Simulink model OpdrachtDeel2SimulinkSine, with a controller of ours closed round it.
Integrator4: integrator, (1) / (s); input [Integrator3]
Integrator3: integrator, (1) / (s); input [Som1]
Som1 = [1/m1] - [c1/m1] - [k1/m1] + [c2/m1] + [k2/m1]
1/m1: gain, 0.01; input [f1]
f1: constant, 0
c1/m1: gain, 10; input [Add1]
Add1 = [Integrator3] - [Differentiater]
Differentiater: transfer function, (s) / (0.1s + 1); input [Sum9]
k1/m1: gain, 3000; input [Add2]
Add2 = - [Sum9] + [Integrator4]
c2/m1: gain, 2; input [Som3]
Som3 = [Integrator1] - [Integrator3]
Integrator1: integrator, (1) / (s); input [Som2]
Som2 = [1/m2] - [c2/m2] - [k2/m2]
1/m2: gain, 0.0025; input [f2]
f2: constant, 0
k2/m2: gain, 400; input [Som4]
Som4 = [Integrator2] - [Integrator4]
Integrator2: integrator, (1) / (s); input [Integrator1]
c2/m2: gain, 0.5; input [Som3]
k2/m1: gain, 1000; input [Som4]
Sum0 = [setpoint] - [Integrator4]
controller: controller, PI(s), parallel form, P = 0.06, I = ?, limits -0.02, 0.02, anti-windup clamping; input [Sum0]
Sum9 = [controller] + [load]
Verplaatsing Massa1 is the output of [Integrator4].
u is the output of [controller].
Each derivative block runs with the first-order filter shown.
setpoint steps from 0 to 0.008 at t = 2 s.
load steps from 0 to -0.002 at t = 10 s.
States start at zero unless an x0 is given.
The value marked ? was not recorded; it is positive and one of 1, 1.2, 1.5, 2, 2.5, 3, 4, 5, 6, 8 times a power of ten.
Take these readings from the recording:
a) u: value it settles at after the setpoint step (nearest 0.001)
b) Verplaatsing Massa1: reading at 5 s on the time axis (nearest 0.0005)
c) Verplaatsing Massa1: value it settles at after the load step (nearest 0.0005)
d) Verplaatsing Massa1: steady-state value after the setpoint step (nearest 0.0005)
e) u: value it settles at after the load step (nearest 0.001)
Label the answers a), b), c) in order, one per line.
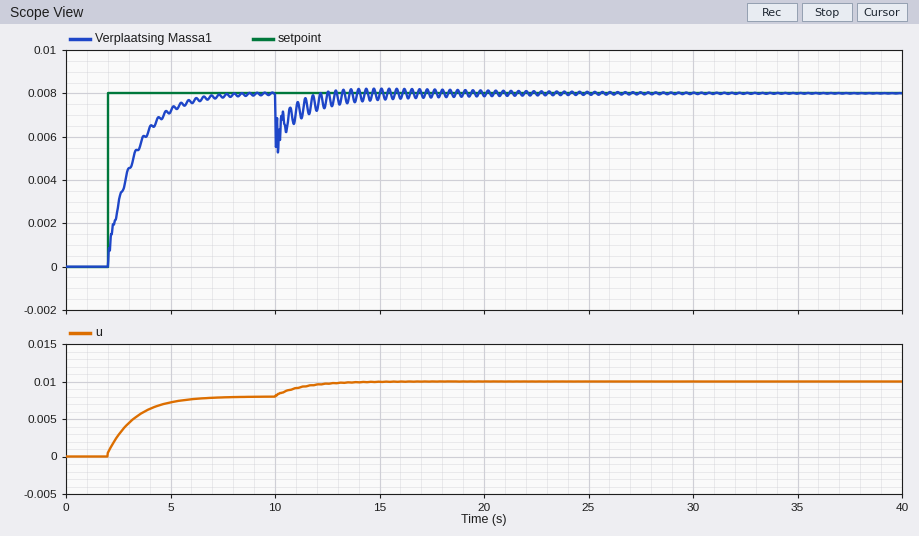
a) 0.008
b) 0.0070
c) 0.0080
d) 0.0080
e) 0.010
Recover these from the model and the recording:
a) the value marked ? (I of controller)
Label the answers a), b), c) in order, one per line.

a) 0.8
